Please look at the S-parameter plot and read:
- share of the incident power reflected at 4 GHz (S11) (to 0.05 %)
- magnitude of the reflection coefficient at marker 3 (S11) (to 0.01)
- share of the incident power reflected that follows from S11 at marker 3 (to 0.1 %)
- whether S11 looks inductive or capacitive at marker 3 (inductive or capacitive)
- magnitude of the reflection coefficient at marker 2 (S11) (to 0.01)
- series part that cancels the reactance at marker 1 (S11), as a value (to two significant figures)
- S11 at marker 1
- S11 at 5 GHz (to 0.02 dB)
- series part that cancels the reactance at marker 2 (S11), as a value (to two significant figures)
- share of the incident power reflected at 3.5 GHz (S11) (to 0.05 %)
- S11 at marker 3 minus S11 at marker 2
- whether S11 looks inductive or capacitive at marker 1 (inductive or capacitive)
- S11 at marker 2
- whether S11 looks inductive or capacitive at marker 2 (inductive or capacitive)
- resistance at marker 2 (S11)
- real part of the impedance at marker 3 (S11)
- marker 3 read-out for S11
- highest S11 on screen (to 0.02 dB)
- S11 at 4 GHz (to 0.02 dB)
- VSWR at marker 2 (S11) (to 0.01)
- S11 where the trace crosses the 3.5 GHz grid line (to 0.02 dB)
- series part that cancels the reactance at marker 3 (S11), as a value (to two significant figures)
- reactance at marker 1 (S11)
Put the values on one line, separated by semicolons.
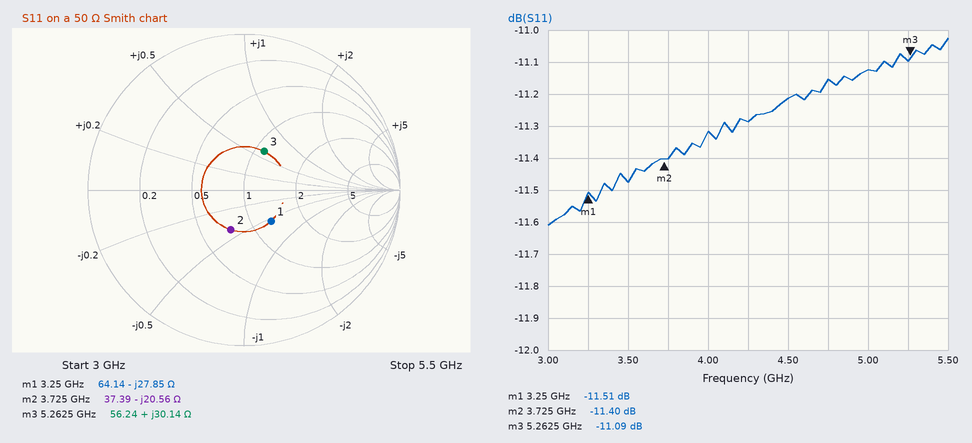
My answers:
7.40 %; 0.28; 7.8 %; inductive; 0.27; 1.4 nH; -11.51 dB; -11.12 dB; 880 pH; 7.10 %; 0.31 dB; capacitive; -11.40 dB; capacitive; 37.39 Ω; 56.24 Ω; -11.09 dB; -11.02 dB; -11.32 dB; 1.74; -11.48 dB; 1.0 pF; -27.85 Ω
